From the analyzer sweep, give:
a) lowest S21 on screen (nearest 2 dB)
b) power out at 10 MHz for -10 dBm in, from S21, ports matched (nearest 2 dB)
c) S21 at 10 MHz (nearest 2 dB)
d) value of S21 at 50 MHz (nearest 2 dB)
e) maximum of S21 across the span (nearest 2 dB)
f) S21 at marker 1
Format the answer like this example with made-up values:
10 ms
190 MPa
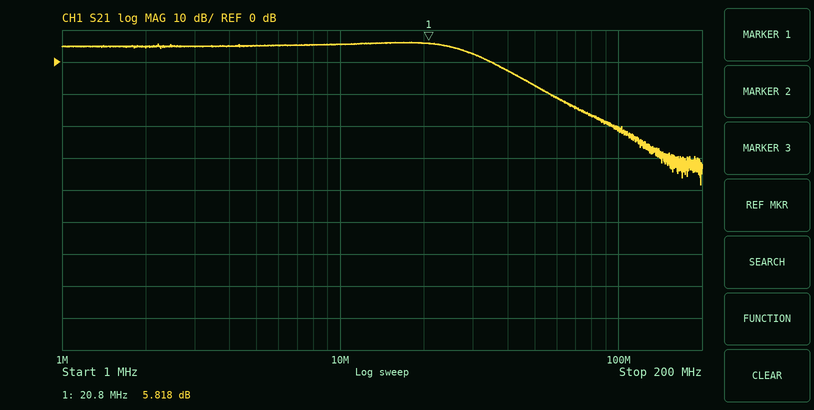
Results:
-38 dB
-4 dBm
6 dB
-8 dB
6 dB
5.818 dB
